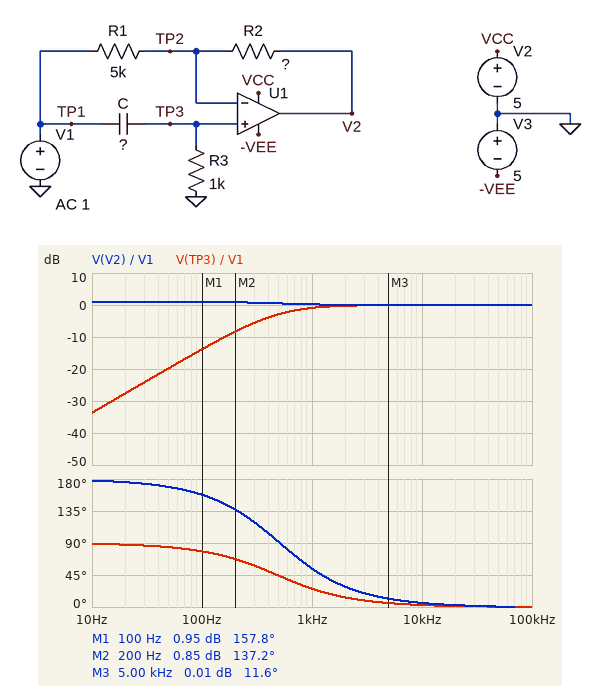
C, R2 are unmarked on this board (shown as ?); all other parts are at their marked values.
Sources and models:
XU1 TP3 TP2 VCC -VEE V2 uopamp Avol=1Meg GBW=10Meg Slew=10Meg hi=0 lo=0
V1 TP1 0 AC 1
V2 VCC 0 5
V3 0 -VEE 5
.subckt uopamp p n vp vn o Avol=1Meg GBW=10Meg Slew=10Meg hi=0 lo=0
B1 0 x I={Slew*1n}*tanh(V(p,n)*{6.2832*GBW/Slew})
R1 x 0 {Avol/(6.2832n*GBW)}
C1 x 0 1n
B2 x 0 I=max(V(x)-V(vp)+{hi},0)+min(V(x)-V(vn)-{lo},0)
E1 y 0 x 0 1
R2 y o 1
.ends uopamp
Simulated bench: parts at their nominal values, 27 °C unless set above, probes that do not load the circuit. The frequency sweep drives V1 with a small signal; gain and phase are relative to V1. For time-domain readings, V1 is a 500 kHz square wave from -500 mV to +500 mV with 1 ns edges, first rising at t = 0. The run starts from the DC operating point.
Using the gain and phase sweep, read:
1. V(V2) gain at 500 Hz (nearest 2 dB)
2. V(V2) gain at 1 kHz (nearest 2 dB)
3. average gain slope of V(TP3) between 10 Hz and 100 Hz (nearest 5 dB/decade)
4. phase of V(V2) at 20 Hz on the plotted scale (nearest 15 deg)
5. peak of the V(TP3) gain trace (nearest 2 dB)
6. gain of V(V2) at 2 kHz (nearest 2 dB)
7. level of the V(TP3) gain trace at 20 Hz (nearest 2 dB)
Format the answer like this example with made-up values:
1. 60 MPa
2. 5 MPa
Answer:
1. 0 dB
2. 0 dB
3. 20 dB/decade
4. 180 deg
5. 0 dB
6. 0 dB
7. -28 dB
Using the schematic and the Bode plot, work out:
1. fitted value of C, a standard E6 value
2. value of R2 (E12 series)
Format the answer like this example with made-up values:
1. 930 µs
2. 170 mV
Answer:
1. 330 nF
2. 5.6 kΩ
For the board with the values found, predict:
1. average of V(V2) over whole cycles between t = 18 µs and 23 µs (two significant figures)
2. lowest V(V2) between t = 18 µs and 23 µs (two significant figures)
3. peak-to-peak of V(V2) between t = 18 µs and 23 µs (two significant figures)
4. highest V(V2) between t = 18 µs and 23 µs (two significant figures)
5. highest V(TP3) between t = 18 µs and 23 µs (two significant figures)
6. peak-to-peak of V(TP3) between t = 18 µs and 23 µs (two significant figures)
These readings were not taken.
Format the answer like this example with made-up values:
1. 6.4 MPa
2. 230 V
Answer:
1. 1.0 V
2. 490 mV
3. 1.0 V
4. 1.5 V
5. 970 mV
6. 1.0 V
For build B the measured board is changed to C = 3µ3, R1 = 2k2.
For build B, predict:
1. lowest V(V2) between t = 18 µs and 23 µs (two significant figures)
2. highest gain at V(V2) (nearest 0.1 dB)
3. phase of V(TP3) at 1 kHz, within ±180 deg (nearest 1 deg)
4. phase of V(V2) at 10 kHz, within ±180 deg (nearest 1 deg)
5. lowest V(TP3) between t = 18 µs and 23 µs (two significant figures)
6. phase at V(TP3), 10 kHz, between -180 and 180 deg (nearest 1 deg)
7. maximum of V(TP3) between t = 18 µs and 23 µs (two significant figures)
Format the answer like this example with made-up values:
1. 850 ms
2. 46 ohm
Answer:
1. 1.3 V
2. 8.1 dB
3. 3 deg
4. 1 deg
5. -3.3 mV
6. 0 deg
7. 1.0 V
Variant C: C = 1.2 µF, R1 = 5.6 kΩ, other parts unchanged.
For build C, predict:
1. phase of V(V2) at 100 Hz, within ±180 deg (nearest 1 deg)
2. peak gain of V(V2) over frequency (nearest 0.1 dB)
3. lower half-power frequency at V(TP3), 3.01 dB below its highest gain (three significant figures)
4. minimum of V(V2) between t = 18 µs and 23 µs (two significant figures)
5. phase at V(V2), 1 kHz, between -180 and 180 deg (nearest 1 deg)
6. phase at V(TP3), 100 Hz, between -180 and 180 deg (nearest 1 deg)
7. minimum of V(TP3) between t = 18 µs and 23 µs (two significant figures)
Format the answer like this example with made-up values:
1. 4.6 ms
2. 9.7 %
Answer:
1. 106 deg
2. 0 dB
3. 133 Hz
4. 480 mV
5. 15 deg
6. 53 deg
7. -9.1 mV
